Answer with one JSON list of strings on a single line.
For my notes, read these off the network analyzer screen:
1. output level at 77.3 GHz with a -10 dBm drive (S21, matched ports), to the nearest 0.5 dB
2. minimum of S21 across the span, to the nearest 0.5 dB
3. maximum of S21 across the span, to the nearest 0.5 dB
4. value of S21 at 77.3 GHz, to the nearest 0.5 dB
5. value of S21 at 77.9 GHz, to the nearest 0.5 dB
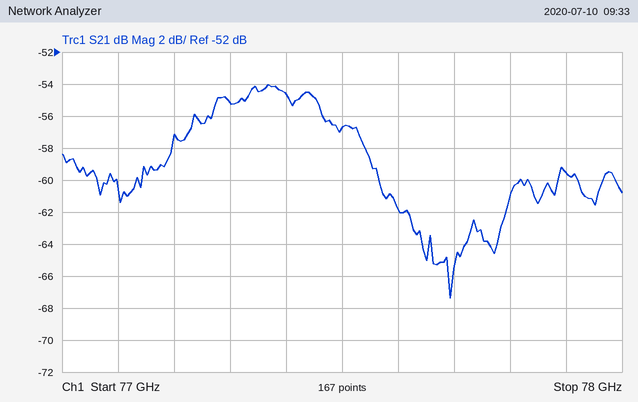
["-65.0 dBm", "-67.5 dB", "-54.0 dB", "-55.0 dB", "-59.5 dB"]
